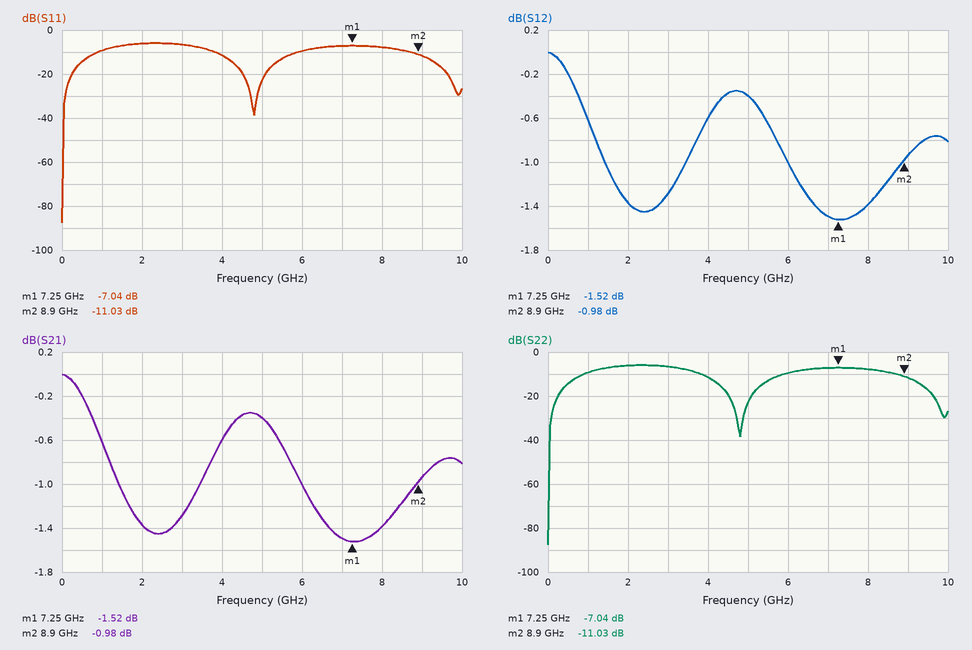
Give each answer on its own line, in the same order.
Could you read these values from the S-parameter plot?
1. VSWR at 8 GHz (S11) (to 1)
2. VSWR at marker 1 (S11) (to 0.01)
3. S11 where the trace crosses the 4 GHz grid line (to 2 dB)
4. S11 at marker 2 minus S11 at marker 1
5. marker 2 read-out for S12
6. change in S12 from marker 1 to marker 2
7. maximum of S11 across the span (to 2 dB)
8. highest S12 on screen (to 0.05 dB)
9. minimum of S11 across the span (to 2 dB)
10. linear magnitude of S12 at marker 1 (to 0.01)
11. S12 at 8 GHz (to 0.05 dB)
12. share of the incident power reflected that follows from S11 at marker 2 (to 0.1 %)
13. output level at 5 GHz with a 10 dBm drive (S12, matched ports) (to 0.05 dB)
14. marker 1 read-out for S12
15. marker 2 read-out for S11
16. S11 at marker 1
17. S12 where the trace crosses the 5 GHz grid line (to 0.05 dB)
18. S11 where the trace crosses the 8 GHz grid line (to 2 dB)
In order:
2
2.60
-12 dB
-3.99 dB
-0.98 dB
0.54 dB
-6 dB
0.00 dB
-88 dB
0.84
-1.40 dB
7.9 %
9.60 dBm
-1.52 dB
-11.03 dB
-7.04 dB
-0.40 dB
-8 dB
